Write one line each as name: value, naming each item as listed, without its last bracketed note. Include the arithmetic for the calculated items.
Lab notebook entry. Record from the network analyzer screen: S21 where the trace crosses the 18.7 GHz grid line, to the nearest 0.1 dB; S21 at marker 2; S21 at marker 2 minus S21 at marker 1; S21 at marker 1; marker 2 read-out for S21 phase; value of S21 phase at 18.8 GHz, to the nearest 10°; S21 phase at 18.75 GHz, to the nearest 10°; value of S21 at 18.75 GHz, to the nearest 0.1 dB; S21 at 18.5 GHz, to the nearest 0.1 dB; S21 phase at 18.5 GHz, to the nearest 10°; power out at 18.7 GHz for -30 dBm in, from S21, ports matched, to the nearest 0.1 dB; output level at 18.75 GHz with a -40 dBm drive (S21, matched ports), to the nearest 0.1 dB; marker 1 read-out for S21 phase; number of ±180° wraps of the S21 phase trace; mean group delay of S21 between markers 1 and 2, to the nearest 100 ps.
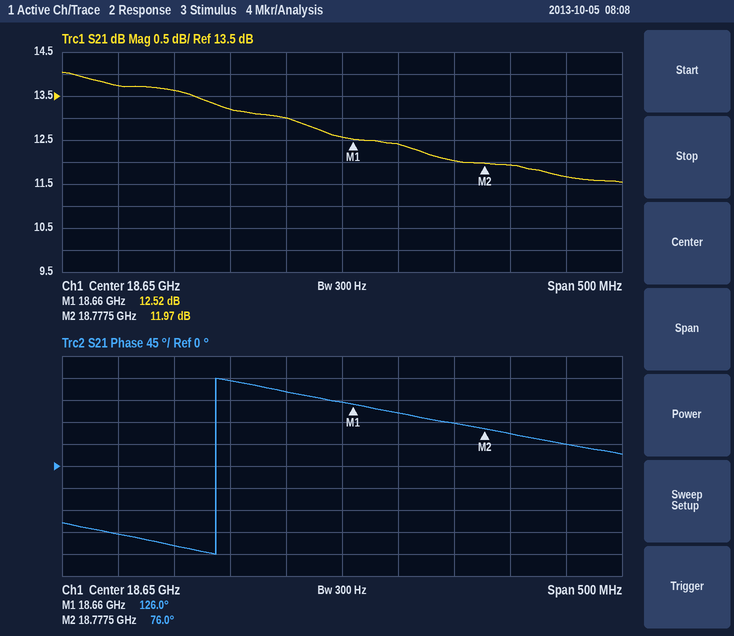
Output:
S21 where the trace crosses the 18.7 GHz grid line, to the nearest 0.1 dB: 12.4 dB
S21 at marker 2: 11.97 dB
S21 at marker 2 minus S21 at marker 1: 11.97 − (12.52) = -0.55 dB
S21 at marker 1: 12.52 dB
marker 2 read-out for S21 phase: 76.0°
value of S21 phase at 18.8 GHz, to the nearest 10°: 70°
S21 phase at 18.75 GHz, to the nearest 10°: 90°
value of S21 at 18.75 GHz, to the nearest 0.1 dB: 12.0 dB
S21 at 18.5 GHz, to the nearest 0.1 dB: 13.6 dB
S21 phase at 18.5 GHz, to the nearest 10°: -160°
power out at 18.7 GHz for -30 dBm in, from S21, ports matched, to the nearest 0.1 dB: -30 dBm + (12.4 dB) = -17.6 dBm
output level at 18.75 GHz with a -40 dBm drive (S21, matched ports), to the nearest 0.1 dB: -40 dBm + (12.0 dB) = -28.0 dBm
marker 1 read-out for S21 phase: 126.0°
number of ±180° wraps of the S21 phase trace: 1
mean group delay of S21 between markers 1 and 2, to the nearest 100 ps: −(76° − (126°))/(360° × 117.5 MHz) ≈ 1.2 ns
